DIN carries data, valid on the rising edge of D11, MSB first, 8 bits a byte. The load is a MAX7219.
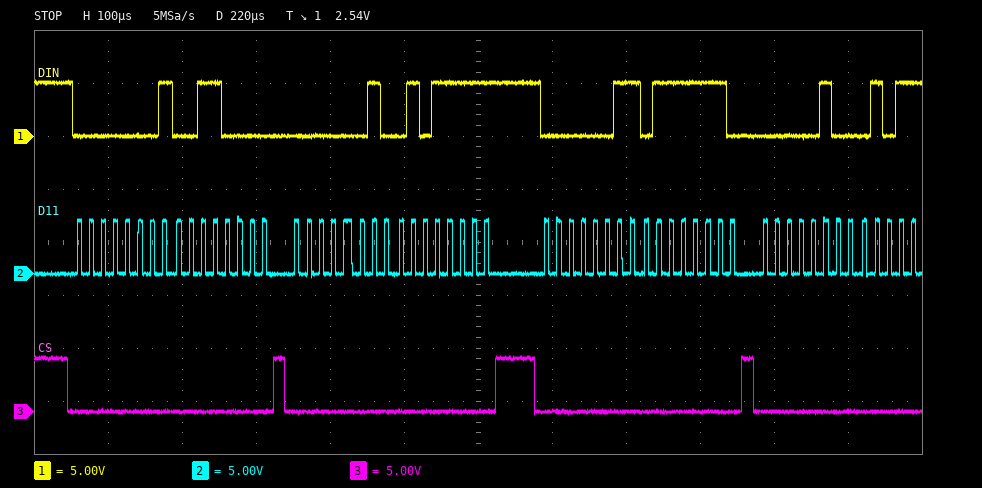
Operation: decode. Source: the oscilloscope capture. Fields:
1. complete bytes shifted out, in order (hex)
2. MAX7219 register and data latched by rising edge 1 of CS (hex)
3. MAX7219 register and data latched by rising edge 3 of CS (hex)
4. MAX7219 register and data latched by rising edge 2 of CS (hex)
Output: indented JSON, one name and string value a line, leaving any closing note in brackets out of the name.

{
  "complete bytes shifted out, in order": "01 30 02 5F 03 7E 04",
  "MAX7219 register and data latched by rising edge 1 of CS": "register 0x1, data 0x30",
  "MAX7219 register and data latched by rising edge 3 of CS": "register 0x3, data 0x7E",
  "MAX7219 register and data latched by rising edge 2 of CS": "register 0x2, data 0x5F"
}
